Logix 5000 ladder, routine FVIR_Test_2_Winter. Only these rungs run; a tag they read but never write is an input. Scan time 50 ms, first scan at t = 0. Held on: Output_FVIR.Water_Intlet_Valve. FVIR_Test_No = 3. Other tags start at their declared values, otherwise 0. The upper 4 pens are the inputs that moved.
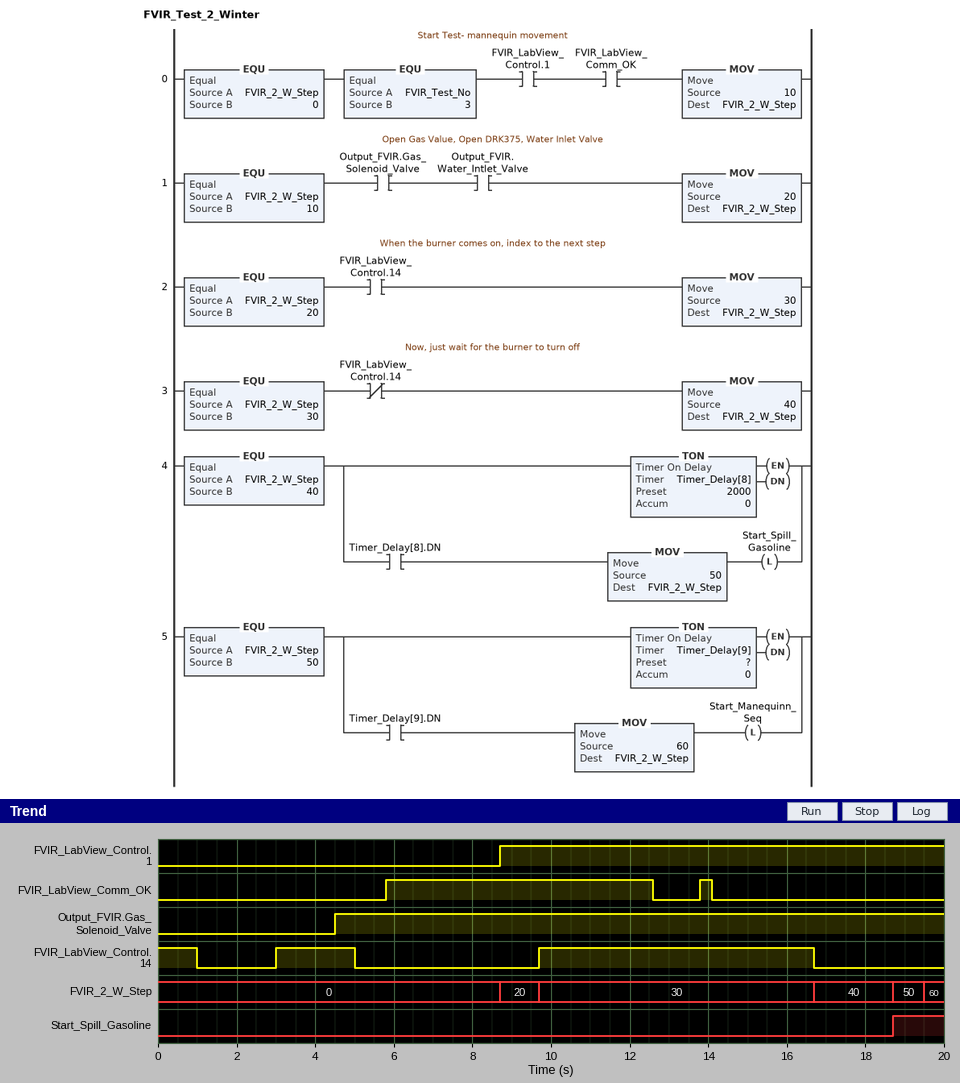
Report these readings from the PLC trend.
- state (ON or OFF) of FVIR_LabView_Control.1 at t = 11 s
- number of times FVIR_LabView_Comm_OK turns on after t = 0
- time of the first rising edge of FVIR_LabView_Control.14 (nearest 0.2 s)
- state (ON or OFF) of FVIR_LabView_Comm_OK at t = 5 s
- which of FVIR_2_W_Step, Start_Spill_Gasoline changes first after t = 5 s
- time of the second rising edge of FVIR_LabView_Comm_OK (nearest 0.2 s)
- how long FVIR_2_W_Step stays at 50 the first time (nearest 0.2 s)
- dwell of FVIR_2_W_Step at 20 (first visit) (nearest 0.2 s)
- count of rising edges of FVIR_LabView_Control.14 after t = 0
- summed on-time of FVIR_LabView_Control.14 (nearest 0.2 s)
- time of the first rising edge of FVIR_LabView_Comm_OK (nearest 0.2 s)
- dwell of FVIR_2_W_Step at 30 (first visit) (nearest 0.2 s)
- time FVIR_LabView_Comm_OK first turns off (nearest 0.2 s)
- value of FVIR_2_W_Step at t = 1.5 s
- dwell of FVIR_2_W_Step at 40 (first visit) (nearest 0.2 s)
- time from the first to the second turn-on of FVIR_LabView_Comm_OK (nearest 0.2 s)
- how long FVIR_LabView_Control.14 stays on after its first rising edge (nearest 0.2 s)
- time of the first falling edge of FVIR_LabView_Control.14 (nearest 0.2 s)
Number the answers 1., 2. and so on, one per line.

1. ON
2. 2
3. 3.0 s
4. OFF
5. FVIR_2_W_Step
6. 13.8 s
7. 0.8 s
8. 1.0 s
9. 2
10. 10.0 s
11. 5.8 s
12. 7.0 s
13. 12.6 s
14. 0
15. 2.0 s
16. 8.0 s
17. 2.0 s
18. 1.0 s
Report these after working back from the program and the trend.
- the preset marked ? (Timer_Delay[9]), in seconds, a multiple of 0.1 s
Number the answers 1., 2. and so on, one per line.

1. 0.8 s
